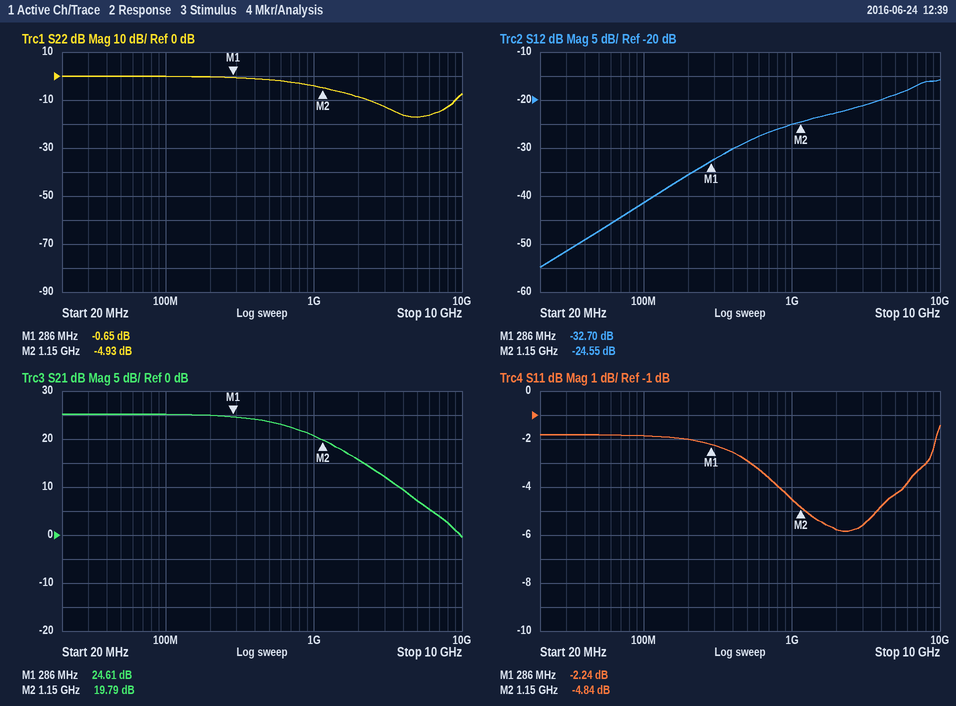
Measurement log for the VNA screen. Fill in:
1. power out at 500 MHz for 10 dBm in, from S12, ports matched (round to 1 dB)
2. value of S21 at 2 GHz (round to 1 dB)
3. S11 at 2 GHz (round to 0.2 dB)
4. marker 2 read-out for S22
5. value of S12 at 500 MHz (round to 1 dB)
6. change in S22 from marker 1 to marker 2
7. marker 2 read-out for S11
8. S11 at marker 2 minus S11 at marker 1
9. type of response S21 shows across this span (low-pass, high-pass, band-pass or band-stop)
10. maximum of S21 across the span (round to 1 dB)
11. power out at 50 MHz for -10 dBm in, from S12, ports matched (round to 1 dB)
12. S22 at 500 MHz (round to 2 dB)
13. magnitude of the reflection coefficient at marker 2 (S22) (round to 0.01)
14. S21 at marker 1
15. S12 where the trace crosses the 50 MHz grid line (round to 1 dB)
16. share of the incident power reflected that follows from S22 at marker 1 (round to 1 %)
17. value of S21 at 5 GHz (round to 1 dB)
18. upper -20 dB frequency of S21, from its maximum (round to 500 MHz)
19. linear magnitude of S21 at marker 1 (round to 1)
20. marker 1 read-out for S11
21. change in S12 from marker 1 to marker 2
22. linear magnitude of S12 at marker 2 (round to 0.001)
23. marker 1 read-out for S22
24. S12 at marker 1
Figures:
-19 dBm
16 dB
-5.8 dB
-4.93 dB
-29 dB
-4.28 dB
-4.84 dB
-2.60 dB
low-pass
25 dB
-57 dBm
-2 dB
0.57
24.61 dB
-47 dB
86 %
7 dB
6.0 GHz
17
-2.24 dB
8.15 dB
0.059
-0.65 dB
-32.70 dB
